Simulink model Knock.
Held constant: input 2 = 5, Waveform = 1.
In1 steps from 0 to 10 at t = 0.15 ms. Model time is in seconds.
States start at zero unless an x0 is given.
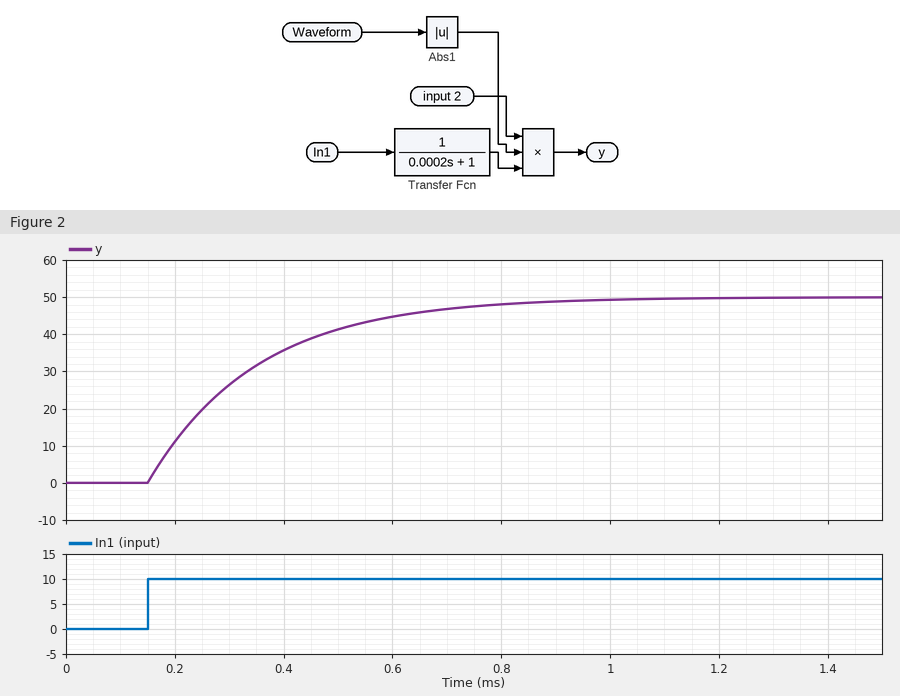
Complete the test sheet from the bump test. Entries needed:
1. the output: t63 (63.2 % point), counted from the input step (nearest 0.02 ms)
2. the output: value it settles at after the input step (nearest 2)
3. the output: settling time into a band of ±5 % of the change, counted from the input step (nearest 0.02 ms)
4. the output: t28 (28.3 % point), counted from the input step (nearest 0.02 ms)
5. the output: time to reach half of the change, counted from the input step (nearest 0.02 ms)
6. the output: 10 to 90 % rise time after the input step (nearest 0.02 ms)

0.20 ms
50
0.60 ms
0.06 ms
0.14 ms
0.44 ms
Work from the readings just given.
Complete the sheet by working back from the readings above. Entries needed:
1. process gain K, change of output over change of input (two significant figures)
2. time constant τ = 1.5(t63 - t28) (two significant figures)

5.0
0.21 ms
